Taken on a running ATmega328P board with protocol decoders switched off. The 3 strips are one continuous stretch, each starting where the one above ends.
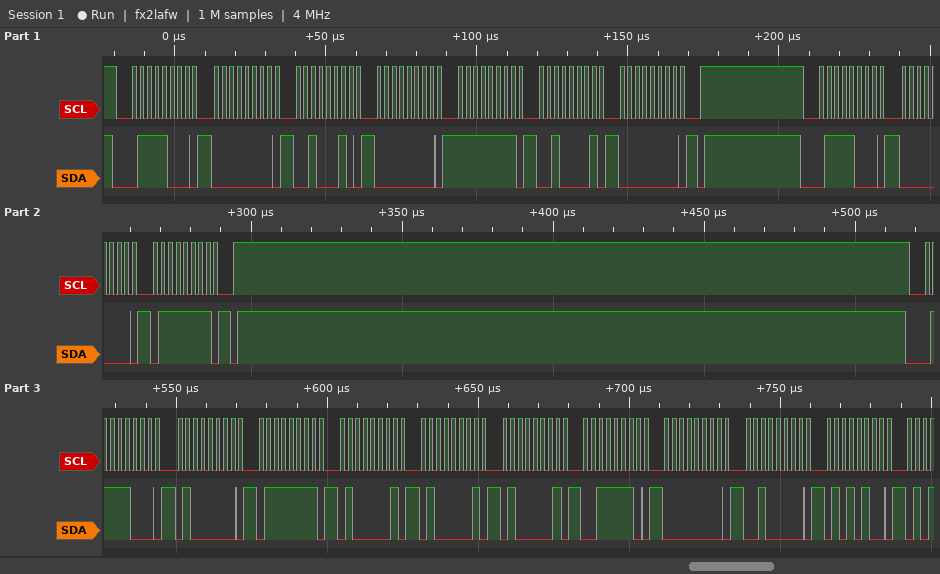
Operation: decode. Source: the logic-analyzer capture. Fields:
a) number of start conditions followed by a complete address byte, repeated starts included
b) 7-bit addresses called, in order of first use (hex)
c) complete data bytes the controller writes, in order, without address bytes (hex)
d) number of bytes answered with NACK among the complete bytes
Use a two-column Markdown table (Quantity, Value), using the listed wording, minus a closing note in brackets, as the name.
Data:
| Quantity | Value |
|---|---|
| number of start conditions followed by a complete address byte, repeated starts included | 3 |
| 7-bit addresses called, in order of first use | 0x3C |
| complete data bytes the controller writes, in order, without address bytes | 00 22 00 FF 21 00 00 7F 40 7F 41 41 41 3E 00 20 54 |
| number of bytes answered with NACK among the complete bytes | 0 |
